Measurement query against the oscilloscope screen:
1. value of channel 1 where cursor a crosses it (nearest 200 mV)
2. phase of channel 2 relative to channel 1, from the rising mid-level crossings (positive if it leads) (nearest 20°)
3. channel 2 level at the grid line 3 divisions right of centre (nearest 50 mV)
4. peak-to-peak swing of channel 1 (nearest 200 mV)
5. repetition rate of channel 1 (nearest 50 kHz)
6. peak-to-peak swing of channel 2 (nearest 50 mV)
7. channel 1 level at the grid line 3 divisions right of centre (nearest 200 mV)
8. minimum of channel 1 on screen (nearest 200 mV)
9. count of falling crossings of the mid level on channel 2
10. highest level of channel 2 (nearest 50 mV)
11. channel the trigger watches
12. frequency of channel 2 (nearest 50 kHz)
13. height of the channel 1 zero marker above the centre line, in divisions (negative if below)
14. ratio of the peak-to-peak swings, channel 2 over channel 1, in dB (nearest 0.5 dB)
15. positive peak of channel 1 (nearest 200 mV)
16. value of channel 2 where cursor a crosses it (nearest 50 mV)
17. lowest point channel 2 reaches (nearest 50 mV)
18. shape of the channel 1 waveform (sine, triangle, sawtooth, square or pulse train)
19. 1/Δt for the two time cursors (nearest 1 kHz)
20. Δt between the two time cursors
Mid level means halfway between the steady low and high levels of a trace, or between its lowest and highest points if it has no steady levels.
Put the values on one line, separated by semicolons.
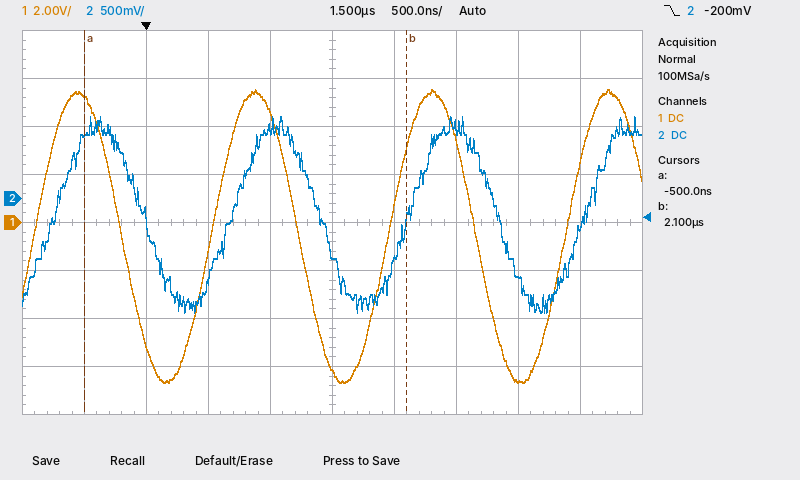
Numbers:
5.2 V; -40°; -800 mV; 12.2 V; 700 kHz; 2.05 V; -6.6 V; -6.6 V; 3; 850 mV; channel 2; 700 kHz; 0.0 div; -15.5 dB; 5.6 V; 650 mV; -1.20 V; sine; 385 kHz; 2.60 µs
